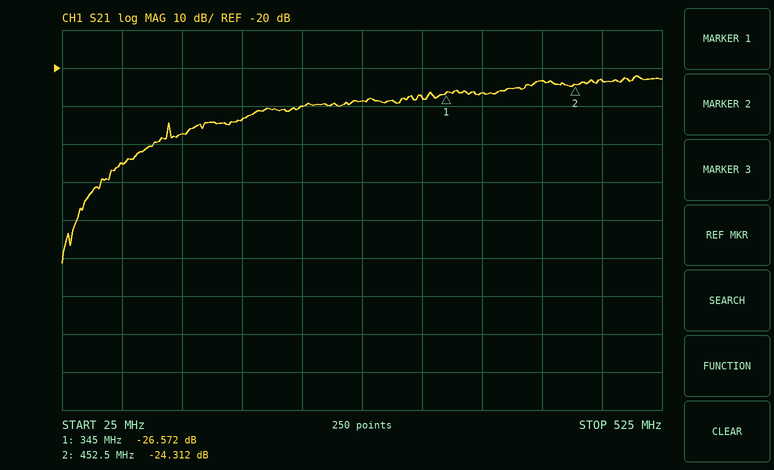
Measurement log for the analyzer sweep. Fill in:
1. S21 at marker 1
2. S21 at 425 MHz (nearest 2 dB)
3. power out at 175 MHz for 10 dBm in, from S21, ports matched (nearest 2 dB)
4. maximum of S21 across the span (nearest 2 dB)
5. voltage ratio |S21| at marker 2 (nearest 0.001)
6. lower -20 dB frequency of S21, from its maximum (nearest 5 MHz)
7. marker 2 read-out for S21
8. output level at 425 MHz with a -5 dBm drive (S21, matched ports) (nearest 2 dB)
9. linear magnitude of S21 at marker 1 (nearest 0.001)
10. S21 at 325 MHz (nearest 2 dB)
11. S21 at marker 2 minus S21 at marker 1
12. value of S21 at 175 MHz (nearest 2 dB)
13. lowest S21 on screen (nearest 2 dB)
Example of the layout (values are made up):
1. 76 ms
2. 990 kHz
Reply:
1. -26.572 dB
2. -24 dB
3. -24 dBm
4. -22 dB
5. 0.061
6. 90 MHz
7. -24.312 dB
8. -28 dBm
9. 0.047
10. -28 dB
11. 2.260 dB
12. -34 dB
13. -72 dB
